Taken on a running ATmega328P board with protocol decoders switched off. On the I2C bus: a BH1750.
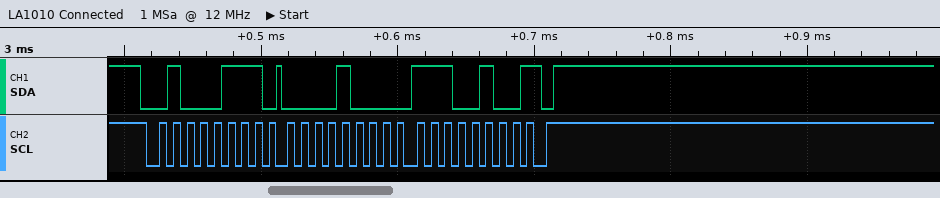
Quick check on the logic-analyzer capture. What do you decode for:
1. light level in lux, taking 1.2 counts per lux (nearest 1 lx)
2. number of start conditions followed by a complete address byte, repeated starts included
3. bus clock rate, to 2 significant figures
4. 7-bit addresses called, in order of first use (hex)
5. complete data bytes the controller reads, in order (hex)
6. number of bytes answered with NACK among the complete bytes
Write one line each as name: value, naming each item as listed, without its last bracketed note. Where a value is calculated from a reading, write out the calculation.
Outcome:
light level in lux, taking 1.2 counts per lux: 2276 / 1.2 = 1897 lx
number of start conditions followed by a complete address byte, repeated starts included: 1
bus clock rate, to 2 significant figures: 100 kHz
7-bit addresses called, in order of first use: 0x23
complete data bytes the controller reads, in order: 08 E4
number of bytes answered with NACK among the complete bytes: 1
